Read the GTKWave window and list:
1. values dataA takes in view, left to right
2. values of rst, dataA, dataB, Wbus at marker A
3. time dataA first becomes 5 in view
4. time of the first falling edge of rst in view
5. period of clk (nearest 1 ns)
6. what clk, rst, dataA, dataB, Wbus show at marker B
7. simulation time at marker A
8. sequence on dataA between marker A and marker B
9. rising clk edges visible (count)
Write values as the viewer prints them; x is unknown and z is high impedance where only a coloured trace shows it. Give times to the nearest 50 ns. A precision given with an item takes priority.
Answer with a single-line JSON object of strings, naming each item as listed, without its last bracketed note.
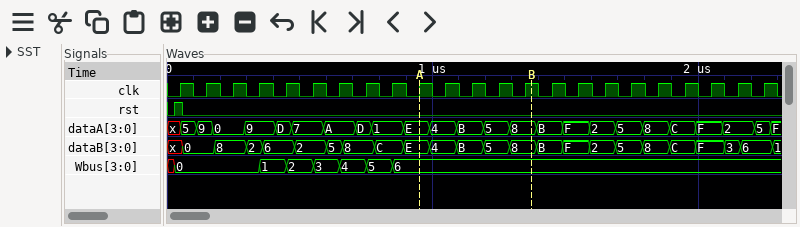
{"values dataA takes in view, left to right": "x, 5, 9, 0, 9, D, 7, A, D, 1, E, 4, B, 5, 8, B, F, 2, 5, 8, C, F, 2, 5, F", "values of rst, dataA, dataB, Wbus at marker A": "rst=0, dataA=E, dataB=E, Wbus=6", "time dataA first becomes 5 in view": "50 ns", "time of the first falling edge of rst in view": "50 ns", "period of clk": "100 ns", "what clk, rst, dataA, dataB, Wbus show at marker B": "clk=1, rst=0, dataA=8, dataB=8, Wbus=6", "simulation time at marker A": "950 ns", "sequence on dataA between marker A and marker B": "E, 4, B, 5, 8", "rising clk edges visible": "23"}
